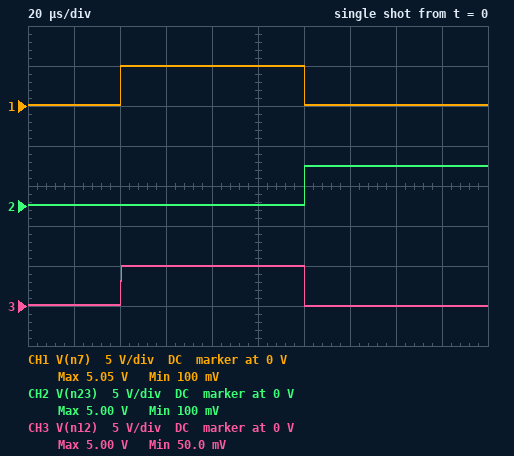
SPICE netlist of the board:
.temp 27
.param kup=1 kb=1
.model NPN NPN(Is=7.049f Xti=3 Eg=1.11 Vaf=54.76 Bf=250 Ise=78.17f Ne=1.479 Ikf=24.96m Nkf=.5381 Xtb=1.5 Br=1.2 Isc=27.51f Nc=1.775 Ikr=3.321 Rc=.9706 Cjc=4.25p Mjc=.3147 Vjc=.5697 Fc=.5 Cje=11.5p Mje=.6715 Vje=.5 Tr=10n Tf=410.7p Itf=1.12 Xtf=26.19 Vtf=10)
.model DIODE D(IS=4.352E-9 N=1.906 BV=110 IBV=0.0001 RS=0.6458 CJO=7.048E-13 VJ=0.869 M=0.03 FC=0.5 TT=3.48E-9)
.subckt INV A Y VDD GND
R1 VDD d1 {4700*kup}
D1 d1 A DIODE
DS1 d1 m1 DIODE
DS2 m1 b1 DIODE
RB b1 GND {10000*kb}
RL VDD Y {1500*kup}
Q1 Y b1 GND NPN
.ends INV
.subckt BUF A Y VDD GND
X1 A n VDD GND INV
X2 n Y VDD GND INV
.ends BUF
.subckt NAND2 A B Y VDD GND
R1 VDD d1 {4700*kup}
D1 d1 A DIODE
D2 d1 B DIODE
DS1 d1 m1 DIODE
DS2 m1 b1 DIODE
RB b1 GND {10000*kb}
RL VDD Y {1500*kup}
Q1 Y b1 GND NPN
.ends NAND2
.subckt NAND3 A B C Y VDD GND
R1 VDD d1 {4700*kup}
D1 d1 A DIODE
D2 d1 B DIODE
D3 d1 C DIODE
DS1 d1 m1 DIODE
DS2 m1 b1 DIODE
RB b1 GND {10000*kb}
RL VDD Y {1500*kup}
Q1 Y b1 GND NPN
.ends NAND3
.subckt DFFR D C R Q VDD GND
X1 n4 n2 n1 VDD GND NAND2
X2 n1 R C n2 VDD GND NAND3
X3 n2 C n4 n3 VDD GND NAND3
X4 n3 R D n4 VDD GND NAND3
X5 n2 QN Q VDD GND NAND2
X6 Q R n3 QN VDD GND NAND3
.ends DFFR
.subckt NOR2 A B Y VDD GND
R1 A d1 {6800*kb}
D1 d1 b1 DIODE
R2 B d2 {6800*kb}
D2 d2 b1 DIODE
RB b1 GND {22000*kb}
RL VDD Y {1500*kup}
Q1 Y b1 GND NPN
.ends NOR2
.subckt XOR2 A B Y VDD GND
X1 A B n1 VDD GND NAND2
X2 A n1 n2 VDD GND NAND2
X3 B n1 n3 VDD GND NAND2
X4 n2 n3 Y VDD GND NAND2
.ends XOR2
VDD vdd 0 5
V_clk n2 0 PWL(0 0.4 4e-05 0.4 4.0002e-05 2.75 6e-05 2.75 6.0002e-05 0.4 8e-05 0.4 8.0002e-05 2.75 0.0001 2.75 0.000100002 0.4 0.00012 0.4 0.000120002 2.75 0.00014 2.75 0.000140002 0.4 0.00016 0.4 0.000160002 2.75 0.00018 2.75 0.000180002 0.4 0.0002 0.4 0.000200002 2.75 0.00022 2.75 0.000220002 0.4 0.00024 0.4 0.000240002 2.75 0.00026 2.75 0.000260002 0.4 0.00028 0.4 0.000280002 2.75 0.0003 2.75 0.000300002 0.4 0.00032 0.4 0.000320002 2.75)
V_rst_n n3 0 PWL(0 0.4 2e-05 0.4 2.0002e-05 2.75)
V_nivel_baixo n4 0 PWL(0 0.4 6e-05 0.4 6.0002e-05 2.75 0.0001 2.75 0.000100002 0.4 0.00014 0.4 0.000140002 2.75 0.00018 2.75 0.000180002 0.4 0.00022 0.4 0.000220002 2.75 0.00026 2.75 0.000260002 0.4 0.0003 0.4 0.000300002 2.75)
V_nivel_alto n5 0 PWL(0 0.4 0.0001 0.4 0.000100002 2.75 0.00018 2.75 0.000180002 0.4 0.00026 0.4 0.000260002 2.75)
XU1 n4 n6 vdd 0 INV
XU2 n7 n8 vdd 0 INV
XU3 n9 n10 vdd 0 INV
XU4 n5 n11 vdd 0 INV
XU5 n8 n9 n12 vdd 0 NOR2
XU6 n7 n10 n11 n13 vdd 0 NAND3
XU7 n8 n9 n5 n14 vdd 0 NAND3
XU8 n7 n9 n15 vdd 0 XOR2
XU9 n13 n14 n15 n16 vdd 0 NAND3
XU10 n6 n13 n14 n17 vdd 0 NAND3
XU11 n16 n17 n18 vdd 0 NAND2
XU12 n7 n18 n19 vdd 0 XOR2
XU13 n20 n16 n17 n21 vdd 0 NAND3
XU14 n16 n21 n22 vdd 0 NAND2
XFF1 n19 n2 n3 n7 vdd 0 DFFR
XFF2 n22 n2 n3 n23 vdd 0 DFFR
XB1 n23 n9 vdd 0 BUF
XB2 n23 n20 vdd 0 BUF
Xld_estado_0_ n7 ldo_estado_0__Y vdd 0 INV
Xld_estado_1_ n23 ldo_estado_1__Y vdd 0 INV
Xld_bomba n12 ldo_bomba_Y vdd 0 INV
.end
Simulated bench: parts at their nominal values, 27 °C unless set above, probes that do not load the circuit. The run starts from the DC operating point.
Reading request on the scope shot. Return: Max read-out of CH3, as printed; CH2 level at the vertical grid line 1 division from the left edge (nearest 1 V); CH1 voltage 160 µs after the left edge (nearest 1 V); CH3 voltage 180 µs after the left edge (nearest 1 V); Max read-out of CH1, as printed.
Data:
5.00 V
0 V
0 V
0 V
5.05 V
